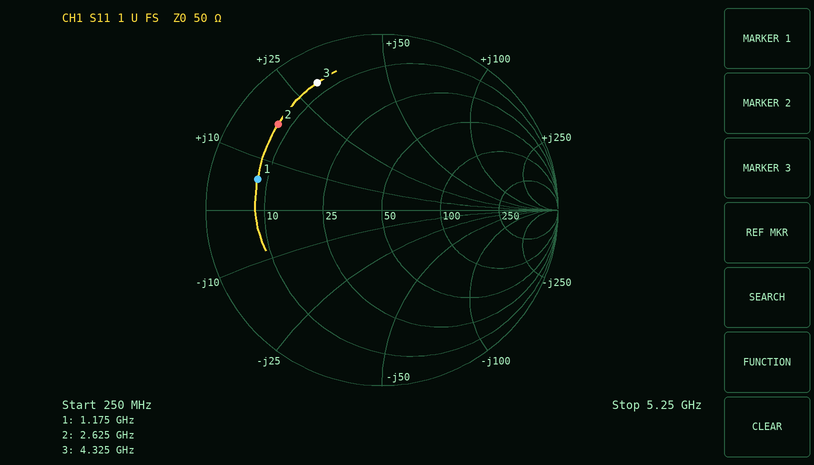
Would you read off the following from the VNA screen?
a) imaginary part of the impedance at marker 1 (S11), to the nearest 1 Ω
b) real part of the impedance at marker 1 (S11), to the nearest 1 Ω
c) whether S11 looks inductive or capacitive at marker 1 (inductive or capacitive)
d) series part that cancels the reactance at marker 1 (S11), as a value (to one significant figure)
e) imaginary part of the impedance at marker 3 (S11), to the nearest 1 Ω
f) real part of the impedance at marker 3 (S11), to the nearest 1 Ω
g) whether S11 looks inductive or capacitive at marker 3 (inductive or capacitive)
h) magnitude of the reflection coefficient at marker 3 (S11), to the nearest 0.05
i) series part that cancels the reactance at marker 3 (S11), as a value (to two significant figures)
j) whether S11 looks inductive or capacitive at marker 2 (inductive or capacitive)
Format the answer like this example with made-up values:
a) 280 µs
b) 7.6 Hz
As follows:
a) +6 Ω
b) 8 Ω
c) inductive
d) 20 pF
e) +30 Ω
f) 7 Ω
g) inductive
h) 0.80
i) 1.2 pF
j) inductive
